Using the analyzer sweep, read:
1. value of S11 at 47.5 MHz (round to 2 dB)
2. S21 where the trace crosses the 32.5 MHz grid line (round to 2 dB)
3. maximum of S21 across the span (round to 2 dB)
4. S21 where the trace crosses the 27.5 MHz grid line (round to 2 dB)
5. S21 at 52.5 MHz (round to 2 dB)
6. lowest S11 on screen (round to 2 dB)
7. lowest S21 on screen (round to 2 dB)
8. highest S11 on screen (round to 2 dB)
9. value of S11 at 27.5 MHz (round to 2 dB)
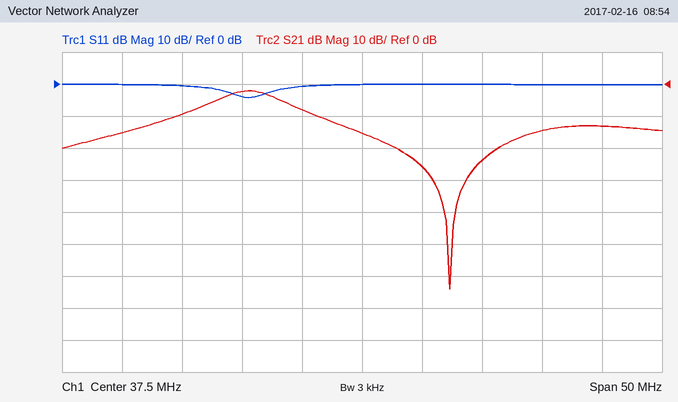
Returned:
0 dB
-8 dB
-2 dB
-2 dB
-14 dB
-4 dB
-64 dB
0 dB
-4 dB
